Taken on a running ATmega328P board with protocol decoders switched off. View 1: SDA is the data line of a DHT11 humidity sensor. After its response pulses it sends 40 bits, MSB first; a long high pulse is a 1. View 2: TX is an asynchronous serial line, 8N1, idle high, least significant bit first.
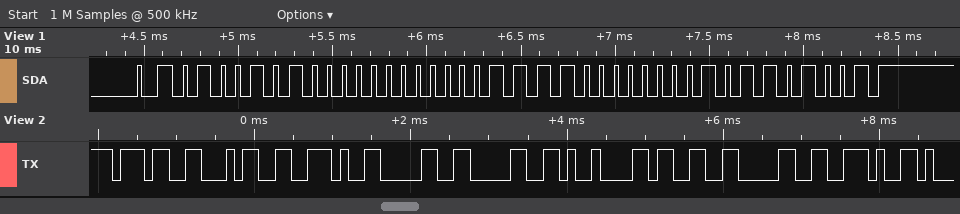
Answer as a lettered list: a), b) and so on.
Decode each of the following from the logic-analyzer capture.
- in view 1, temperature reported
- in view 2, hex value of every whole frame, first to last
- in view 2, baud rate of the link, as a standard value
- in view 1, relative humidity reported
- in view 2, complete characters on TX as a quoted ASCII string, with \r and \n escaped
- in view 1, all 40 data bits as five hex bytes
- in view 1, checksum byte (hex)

a) 30.1 °C
b) 37 34 2E 30 30 09 33 30 2E
c) 9600 baud
d) 74 %
e) "74.00\t30."
f) 4A 00 1E 01 69
g) 0x69
